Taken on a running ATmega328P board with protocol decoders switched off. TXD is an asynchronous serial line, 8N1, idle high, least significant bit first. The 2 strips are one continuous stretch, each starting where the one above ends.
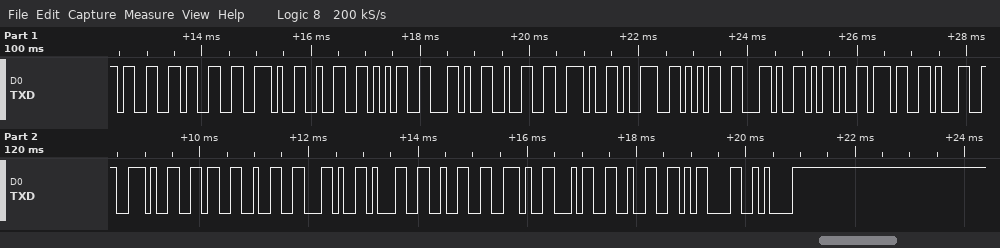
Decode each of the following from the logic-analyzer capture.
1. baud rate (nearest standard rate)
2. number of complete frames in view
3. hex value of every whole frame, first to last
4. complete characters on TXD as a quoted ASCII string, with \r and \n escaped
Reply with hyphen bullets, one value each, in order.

- 9600 baud
- 25
- 33 33 2E 32 35 2C 32 2E 39 35 2C 2D 37 31 2E 36 32 2C 31 32 2E 34 32 0D 0A
- "33.25,2.95,-71.62,12.42\r\n"
